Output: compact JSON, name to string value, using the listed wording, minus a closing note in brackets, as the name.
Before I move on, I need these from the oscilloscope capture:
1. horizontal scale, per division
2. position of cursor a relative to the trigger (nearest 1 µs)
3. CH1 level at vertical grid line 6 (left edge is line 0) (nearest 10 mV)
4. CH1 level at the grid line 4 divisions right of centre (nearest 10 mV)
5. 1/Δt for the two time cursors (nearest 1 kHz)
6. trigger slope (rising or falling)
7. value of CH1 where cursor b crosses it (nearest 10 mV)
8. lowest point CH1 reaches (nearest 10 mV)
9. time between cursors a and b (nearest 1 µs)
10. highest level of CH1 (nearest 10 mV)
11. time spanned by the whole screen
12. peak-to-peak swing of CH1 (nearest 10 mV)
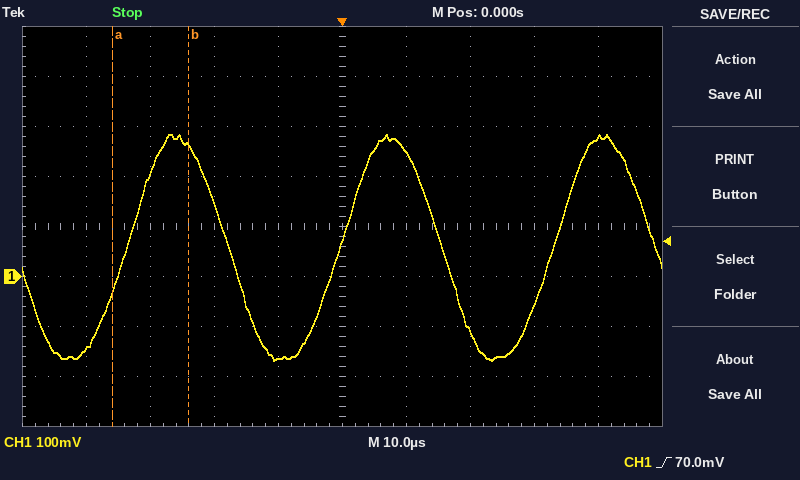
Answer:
{"horizontal scale, per division": "10 µs", "position of cursor a relative to the trigger": "-36 µs", "CH1 level at vertical grid line 6 (left edge is line 0)": "250 mV", "CH1 level at the grid line 4 divisions right of centre": "280 mV", "1/Δt for the two time cursors": "83 kHz", "trigger slope": "rising", "value of CH1 where cursor b crosses it": "260 mV", "lowest point CH1 reaches": "-170 mV", "time between cursors a and b": "12 µs", "highest level of CH1": "280 mV", "time spanned by the whole screen": "100 µs", "peak-to-peak swing of CH1": "450 mV"}
